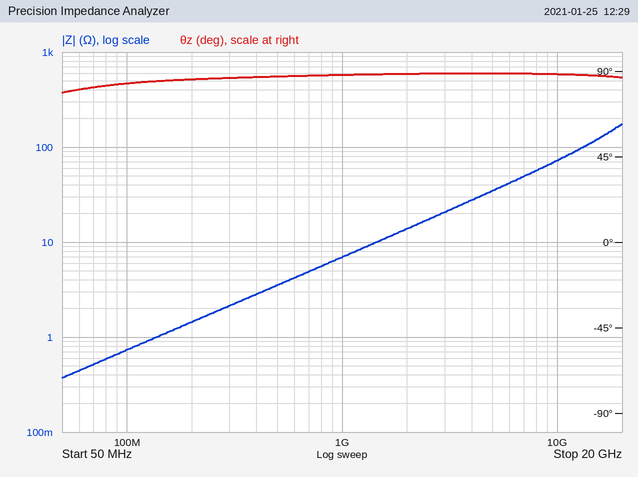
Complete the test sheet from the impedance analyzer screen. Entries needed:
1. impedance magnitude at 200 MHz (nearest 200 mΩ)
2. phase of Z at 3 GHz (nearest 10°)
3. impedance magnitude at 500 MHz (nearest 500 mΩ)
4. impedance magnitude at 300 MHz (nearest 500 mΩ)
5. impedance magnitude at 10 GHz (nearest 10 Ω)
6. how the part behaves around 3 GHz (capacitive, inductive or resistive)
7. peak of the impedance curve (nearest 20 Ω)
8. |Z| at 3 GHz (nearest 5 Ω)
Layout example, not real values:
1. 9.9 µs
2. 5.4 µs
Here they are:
1. 1.4 Ω
2. 90°
3. 3.5 Ω
4. 2.0 Ω
5. 70 Ω
6. inductive
7. 180 Ω
8. 20 Ω
